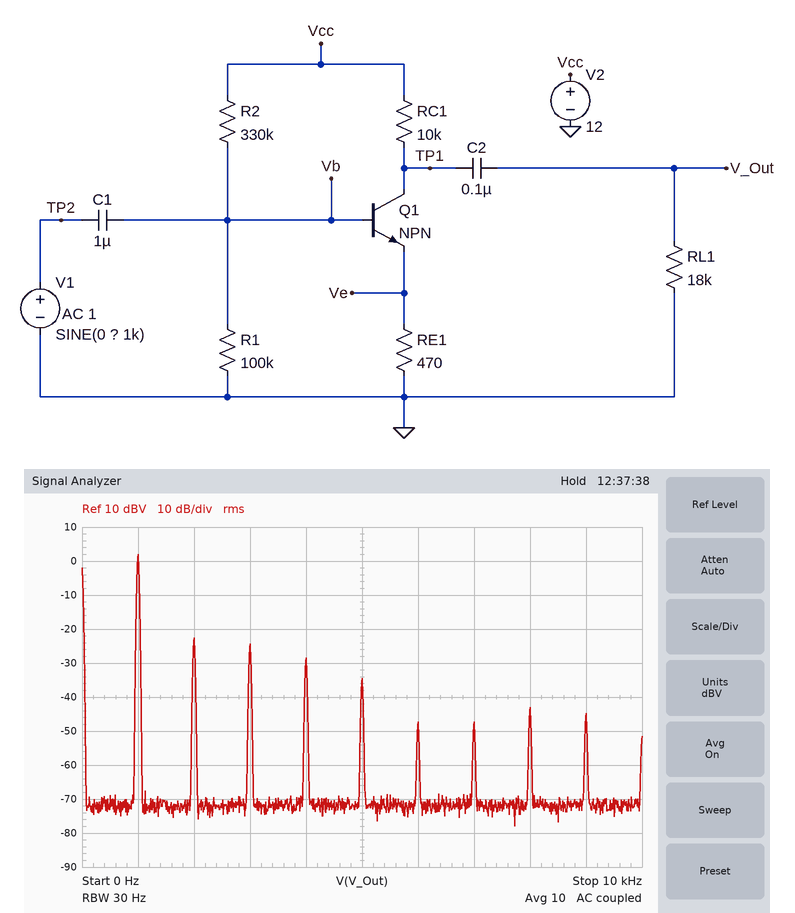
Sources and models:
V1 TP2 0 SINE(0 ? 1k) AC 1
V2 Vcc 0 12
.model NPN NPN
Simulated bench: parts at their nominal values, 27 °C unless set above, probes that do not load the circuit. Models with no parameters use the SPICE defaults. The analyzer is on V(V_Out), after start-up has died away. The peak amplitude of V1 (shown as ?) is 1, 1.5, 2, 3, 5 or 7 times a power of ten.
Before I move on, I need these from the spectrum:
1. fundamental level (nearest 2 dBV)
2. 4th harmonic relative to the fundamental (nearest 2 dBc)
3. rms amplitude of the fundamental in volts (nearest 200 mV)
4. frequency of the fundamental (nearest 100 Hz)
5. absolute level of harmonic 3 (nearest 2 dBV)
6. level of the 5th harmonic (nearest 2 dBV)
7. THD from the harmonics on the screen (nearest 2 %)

2 dBV
-30 dBc
1.2 V
1.0 kHz
-24 dBV
-34 dBV
8 %
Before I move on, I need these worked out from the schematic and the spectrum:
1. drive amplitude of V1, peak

150 mV
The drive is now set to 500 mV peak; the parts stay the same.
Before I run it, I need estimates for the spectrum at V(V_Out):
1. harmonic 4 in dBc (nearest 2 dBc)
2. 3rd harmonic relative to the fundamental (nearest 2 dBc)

-42 dBc
-20 dBc
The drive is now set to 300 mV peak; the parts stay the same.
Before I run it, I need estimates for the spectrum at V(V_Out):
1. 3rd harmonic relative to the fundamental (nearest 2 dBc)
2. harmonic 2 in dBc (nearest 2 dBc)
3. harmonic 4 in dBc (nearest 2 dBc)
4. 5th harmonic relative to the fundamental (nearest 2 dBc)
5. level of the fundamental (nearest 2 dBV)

-28 dBc
-32 dBc
-32 dBc
-36 dBc
8 dBV
